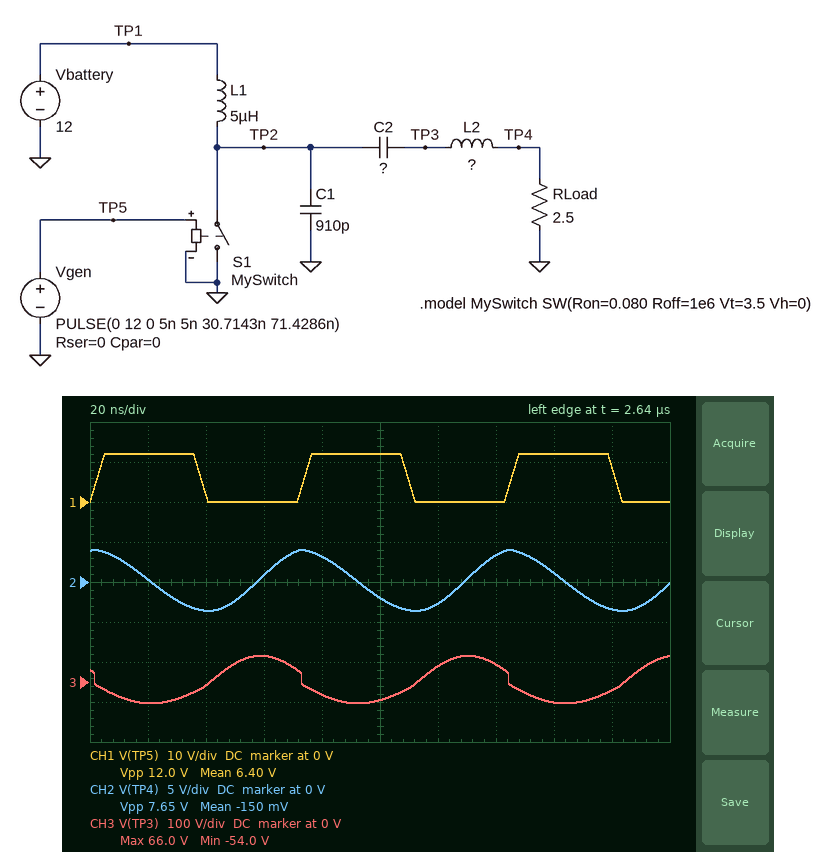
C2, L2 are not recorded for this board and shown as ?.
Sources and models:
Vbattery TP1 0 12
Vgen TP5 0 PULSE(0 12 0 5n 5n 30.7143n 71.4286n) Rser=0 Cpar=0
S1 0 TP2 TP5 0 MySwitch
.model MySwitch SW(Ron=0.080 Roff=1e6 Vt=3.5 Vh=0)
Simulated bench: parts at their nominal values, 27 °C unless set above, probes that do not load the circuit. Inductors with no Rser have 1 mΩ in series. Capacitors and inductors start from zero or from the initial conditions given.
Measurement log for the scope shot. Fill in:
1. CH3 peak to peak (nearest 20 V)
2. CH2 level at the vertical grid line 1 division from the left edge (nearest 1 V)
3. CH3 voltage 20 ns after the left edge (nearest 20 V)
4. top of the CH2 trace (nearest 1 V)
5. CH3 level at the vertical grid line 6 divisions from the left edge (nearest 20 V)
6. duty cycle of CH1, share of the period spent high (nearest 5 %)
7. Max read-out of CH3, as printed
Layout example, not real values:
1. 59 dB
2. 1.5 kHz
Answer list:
1. 120 V
2. 0 V
3. -60 V
4. 4 V
5. 40 V
6. 50 %
7. 66.0 V
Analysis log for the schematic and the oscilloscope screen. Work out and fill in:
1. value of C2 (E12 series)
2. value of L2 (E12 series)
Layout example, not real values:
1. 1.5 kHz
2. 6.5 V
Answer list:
1. 390 pF
2. 470 nH
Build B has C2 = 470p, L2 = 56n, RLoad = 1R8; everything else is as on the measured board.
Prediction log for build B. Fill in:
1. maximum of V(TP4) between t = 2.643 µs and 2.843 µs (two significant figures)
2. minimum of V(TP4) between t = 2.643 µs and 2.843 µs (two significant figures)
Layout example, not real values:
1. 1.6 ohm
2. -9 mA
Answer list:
1. 3.9 V
2. -4.7 V
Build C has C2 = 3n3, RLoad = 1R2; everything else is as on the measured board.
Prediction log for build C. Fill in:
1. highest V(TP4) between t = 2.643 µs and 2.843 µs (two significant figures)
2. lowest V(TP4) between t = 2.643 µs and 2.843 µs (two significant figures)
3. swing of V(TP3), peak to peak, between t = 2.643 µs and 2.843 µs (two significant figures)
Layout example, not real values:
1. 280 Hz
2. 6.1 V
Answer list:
1. 780 mV
2. -580 mV
3. 45 V
